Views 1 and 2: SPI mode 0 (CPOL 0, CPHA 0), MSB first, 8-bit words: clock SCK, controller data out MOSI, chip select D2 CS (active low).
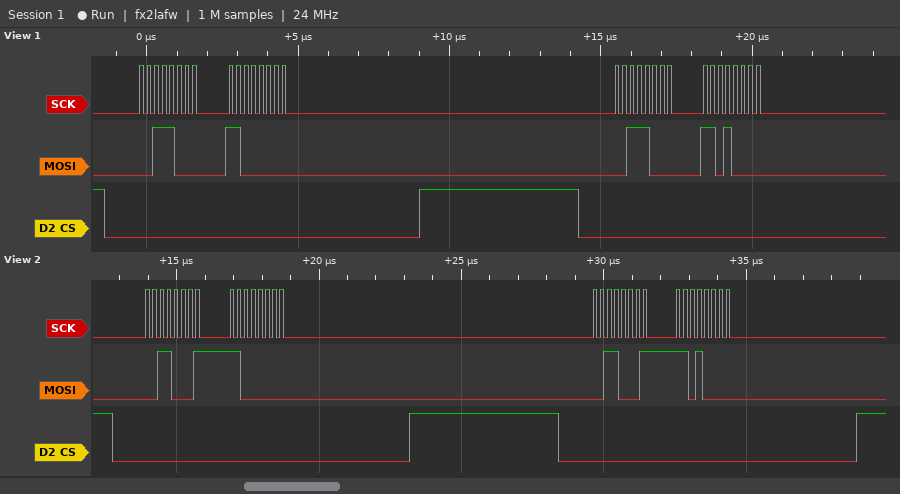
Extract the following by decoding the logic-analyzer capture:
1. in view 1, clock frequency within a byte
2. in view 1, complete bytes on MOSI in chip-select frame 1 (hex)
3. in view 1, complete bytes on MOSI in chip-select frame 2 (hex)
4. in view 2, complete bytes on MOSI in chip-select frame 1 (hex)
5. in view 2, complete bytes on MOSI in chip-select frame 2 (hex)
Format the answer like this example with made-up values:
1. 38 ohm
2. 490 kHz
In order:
1. 4 MHz
2. 38 C0
3. 38 D0
4. 31 C0
5. 31 D0
